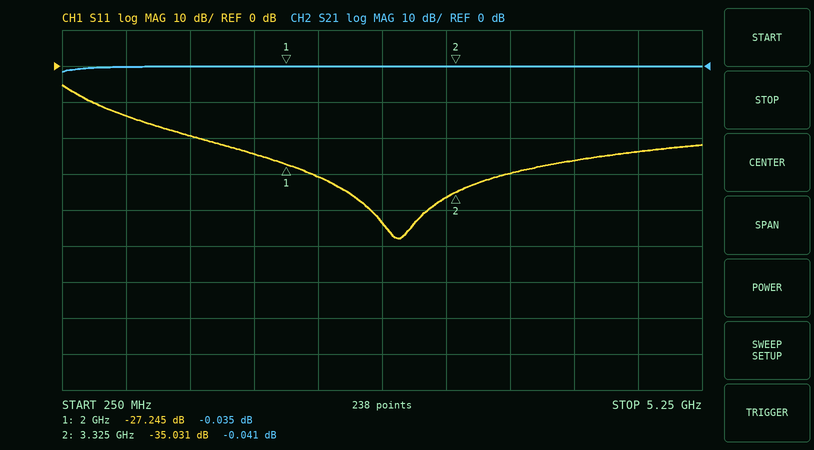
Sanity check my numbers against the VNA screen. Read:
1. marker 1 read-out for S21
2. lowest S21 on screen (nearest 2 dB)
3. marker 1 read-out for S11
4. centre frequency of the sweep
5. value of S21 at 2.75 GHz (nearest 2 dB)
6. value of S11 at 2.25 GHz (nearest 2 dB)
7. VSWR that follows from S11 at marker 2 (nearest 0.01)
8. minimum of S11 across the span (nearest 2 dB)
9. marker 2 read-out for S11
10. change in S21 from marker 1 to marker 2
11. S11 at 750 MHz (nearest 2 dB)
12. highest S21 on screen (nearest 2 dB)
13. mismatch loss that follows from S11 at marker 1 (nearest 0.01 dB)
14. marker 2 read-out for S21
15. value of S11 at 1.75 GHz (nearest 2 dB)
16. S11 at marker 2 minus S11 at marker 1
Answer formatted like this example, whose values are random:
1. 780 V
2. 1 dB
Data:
1. -0.035 dB
2. -2 dB
3. -27.245 dB
4. 2.75 GHz
5. 0 dB
6. -30 dB
7. 1.04
8. -48 dB
9. -35.031 dB
10. -0.006 dB
11. -14 dB
12. 0 dB
13. 0.01 dB
14. -0.041 dB
15. -24 dB
16. -7.786 dB
